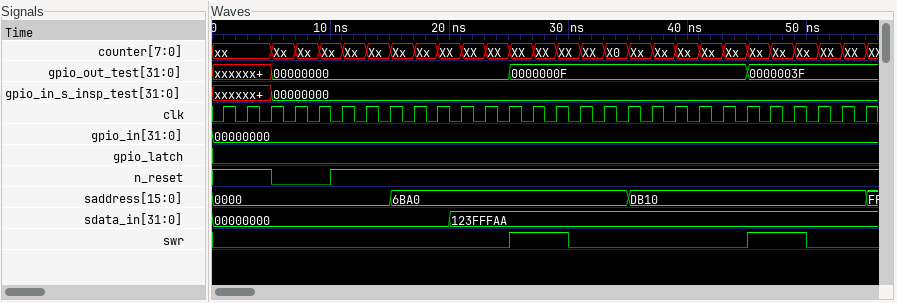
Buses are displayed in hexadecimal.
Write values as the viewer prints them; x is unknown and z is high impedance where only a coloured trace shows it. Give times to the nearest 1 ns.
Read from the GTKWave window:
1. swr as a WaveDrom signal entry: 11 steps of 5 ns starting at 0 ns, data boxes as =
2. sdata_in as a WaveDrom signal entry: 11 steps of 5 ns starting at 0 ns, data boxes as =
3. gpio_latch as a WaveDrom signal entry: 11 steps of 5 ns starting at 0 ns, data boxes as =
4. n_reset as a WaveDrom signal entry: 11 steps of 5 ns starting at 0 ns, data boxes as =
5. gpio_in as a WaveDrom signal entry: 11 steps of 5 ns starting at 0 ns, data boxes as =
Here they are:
{name: 'swr', wave: '0....10..10'}
{name: 'sdata_in', wave: '=...=......', data: '00000000 123FFFAA'}
{name: 'gpio_latch', wave: '0..........'}
{name: 'n_reset', wave: '101........'}
{name: 'gpio_in', wave: '=..........', data: '00000000'}
